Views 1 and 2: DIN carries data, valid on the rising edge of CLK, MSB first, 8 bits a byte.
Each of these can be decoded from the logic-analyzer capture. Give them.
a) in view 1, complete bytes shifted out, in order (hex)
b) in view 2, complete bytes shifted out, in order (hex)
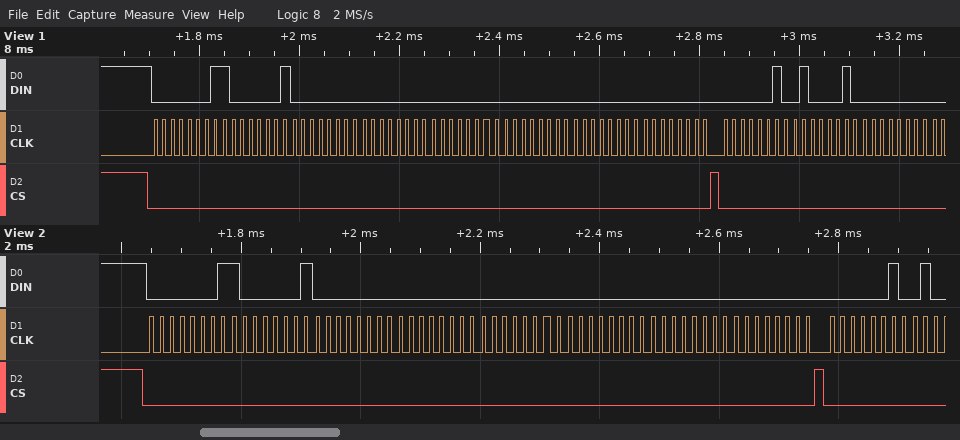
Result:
01 81 00 00 00 00 00 00 02 42 00
01 81 00 00 00 00 00 00 02
